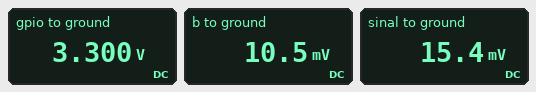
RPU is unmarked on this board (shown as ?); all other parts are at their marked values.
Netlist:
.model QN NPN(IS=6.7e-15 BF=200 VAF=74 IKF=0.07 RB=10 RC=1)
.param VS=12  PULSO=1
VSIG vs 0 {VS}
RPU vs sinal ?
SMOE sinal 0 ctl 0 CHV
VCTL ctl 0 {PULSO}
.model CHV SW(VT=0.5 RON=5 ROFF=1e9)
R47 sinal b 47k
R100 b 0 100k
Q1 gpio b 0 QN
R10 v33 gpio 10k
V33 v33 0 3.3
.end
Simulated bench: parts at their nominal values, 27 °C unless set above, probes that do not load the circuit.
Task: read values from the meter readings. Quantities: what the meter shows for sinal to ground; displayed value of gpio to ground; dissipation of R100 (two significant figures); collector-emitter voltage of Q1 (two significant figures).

15.4 mV
3.300 V
1.1 nW
3.3 V
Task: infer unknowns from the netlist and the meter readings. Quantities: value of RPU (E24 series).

3.9 kΩ
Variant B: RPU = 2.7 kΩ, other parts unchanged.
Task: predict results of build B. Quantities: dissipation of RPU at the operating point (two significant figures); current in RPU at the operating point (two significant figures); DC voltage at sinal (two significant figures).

53 mW
4.4 mA
22 mV
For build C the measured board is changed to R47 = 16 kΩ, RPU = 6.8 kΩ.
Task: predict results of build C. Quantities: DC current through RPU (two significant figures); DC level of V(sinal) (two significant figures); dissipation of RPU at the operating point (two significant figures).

1.8 mA
8.8 mV
21 mW
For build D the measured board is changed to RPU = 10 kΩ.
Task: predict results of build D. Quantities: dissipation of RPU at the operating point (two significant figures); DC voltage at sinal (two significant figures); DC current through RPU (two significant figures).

14 mW
6.0 mV
1.2 mA
